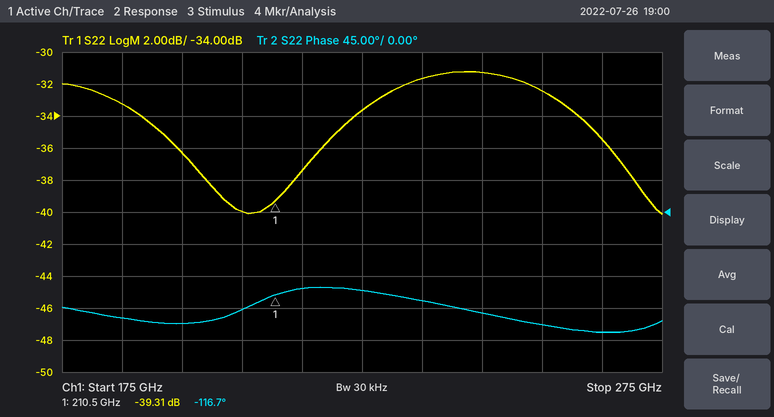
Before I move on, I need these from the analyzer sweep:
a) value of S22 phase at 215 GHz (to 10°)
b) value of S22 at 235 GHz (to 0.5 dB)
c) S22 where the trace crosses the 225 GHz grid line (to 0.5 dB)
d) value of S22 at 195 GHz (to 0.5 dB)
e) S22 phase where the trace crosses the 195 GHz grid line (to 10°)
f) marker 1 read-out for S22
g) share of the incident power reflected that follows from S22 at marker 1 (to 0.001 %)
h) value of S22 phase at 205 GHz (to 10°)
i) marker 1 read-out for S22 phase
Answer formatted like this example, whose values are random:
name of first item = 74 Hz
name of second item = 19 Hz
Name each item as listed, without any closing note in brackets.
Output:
value of S22 phase at 215 GHz = -110°
value of S22 at 235 GHz = -31.5 dB
S22 where the trace crosses the 225 GHz grid line = -33.5 dB
value of S22 at 195 GHz = -36.5 dB
S22 phase where the trace crosses the 195 GHz grid line = -160°
marker 1 read-out for S22 = -39.31 dB
share of the incident power reflected that follows from S22 at marker 1 = 0.012 %
value of S22 phase at 205 GHz = -140°
marker 1 read-out for S22 phase = -116.7°
